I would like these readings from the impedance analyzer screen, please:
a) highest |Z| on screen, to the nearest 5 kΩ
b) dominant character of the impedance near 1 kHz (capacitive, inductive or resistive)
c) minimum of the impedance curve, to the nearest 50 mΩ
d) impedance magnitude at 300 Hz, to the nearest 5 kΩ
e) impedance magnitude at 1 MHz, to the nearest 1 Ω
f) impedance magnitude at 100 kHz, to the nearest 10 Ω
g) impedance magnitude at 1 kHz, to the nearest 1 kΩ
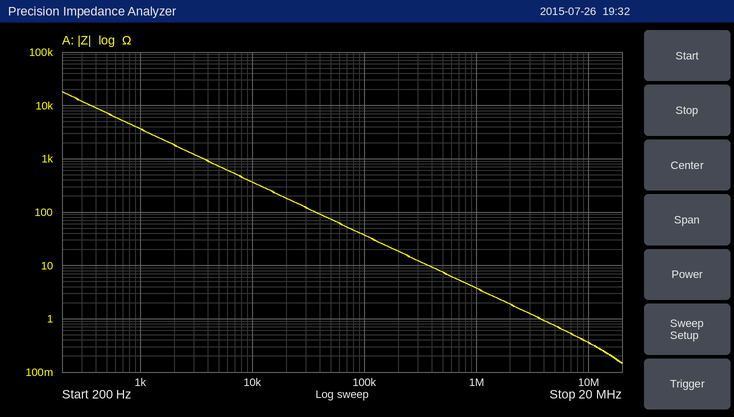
20 kΩ
capacitive
150 mΩ
10 kΩ
4 Ω
40 Ω
4 kΩ
